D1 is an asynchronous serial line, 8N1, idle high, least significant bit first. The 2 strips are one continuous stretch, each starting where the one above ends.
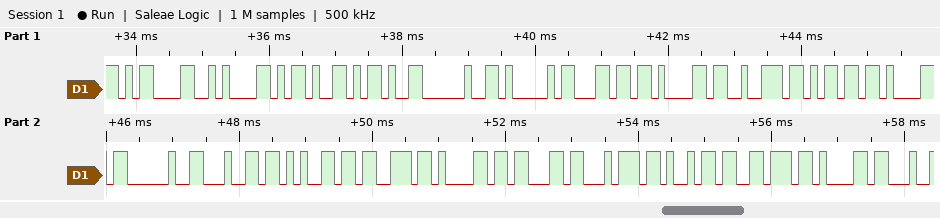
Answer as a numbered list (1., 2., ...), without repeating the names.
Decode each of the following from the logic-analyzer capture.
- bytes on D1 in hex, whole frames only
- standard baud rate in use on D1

1. 0D 0A 2D 2D 20 41 6C 61 72 6D 61 20 64 65 73 61 63 74 69 76 61
2. 9600 baud
